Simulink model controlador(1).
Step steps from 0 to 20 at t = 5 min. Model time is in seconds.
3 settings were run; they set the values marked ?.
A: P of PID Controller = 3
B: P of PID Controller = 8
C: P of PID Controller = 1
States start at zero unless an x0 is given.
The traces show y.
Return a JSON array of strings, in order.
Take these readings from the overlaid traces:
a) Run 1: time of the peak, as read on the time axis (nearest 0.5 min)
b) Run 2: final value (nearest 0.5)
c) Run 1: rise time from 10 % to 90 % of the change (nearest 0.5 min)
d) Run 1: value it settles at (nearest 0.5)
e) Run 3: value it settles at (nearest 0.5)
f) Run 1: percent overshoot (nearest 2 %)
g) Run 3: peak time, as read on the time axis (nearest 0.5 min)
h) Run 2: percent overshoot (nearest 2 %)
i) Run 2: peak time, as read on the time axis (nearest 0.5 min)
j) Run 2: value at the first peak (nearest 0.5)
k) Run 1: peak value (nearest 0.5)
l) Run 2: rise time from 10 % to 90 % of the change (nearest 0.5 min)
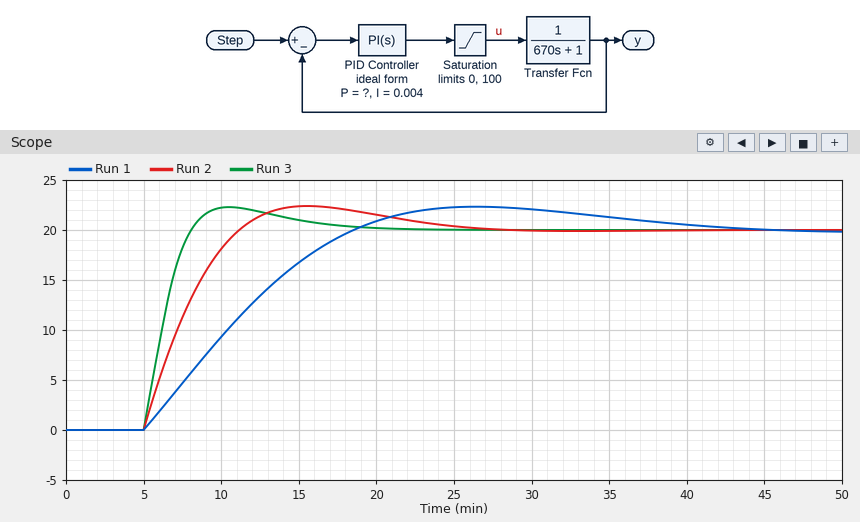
["26.5 min", "20.0", "10.0 min", "20.0", "20.0", "12 %", "10.5 min", "12 %", "15.5 min", "22.5", "22.5", "4.5 min"]
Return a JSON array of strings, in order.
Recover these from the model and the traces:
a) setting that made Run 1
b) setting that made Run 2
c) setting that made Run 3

["C", "A", "B"]
